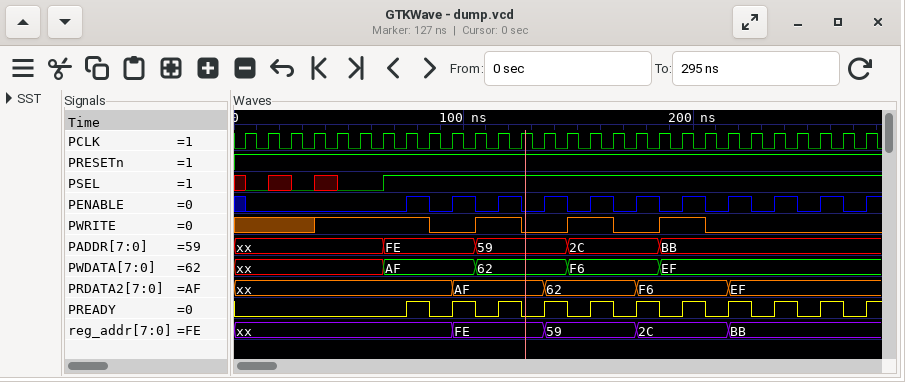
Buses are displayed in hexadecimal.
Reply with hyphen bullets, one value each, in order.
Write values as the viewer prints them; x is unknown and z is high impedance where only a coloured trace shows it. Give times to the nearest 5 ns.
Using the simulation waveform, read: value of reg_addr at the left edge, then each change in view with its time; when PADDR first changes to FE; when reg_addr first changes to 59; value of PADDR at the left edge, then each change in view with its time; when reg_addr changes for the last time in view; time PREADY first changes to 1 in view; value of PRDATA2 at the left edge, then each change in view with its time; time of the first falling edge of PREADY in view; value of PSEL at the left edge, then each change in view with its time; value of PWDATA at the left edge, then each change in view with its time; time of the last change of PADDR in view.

- xx, FE at 95 ns, 59 at 135 ns, 2C at 175 ns, BB at 215 ns
- 65 ns
- 135 ns
- xx, FE at 65 ns, 59 at 105 ns, 2C at 145 ns, BB at 185 ns
- 215 ns
- 75 ns
- xx, AF at 95 ns, 62 at 135 ns, F6 at 175 ns, EF at 215 ns
- 85 ns
- x, 0 at 5 ns, x at 15 ns, 0 at 25 ns, x at 35 ns, 0 at 45 ns, 1 at 65 ns
- xx, AF at 65 ns, 62 at 105 ns, F6 at 145 ns, EF at 185 ns
- 185 ns
